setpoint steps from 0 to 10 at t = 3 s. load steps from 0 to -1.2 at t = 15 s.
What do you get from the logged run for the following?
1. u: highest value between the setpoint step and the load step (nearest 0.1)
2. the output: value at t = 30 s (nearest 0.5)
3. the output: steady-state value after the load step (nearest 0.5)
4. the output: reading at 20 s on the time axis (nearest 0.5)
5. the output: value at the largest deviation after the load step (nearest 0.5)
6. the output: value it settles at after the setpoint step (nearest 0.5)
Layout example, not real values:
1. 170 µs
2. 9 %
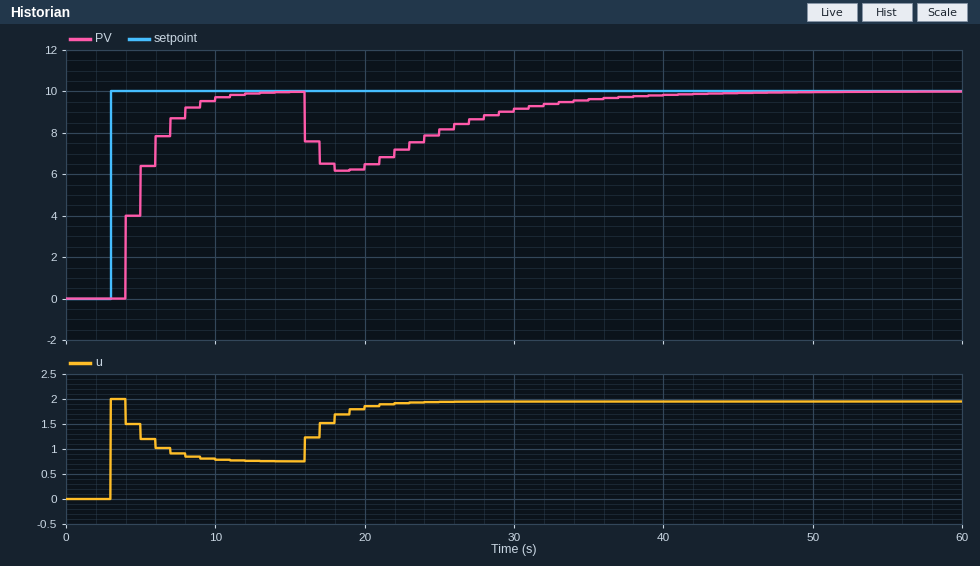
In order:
1. 2.0
2. 9.0
3. 10.0
4. 6.5
5. 6.0
6. 10.0
